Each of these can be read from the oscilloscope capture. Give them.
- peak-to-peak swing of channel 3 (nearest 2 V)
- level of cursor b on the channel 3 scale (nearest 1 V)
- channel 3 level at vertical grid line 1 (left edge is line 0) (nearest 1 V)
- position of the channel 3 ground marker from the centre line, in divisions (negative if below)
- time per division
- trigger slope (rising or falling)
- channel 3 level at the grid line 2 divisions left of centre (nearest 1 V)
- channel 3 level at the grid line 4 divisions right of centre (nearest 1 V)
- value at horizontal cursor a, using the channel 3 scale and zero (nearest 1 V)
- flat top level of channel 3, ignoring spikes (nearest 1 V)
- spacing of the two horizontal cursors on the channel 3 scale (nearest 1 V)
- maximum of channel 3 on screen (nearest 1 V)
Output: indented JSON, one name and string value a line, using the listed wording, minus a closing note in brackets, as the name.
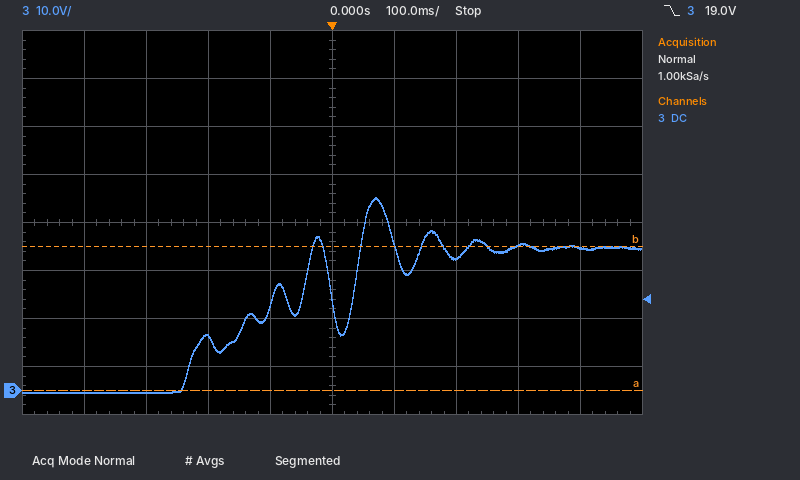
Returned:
{
  "peak-to-peak swing of channel 3": "40 V",
  "level of cursor b on the channel 3 scale": "30 V",
  "channel 3 level at vertical grid line 1 (left edge is line 0)": "0 V",
  "position of the channel 3 ground marker from the centre line, in divisions": "-3.5 div",
  "time per division": "100 ms",
  "trigger slope": "falling",
  "channel 3 level at the grid line 2 divisions left of centre": "11 V",
  "channel 3 level at the grid line 4 divisions right of centre": "30 V",
  "value at horizontal cursor a, using the channel 3 scale and zero": "0 V",
  "flat top level of channel 3, ignoring spikes": "30 V",
  "spacing of the two horizontal cursors on the channel 3 scale": "30 V",
  "maximum of channel 3 on screen": "40 V"
}
